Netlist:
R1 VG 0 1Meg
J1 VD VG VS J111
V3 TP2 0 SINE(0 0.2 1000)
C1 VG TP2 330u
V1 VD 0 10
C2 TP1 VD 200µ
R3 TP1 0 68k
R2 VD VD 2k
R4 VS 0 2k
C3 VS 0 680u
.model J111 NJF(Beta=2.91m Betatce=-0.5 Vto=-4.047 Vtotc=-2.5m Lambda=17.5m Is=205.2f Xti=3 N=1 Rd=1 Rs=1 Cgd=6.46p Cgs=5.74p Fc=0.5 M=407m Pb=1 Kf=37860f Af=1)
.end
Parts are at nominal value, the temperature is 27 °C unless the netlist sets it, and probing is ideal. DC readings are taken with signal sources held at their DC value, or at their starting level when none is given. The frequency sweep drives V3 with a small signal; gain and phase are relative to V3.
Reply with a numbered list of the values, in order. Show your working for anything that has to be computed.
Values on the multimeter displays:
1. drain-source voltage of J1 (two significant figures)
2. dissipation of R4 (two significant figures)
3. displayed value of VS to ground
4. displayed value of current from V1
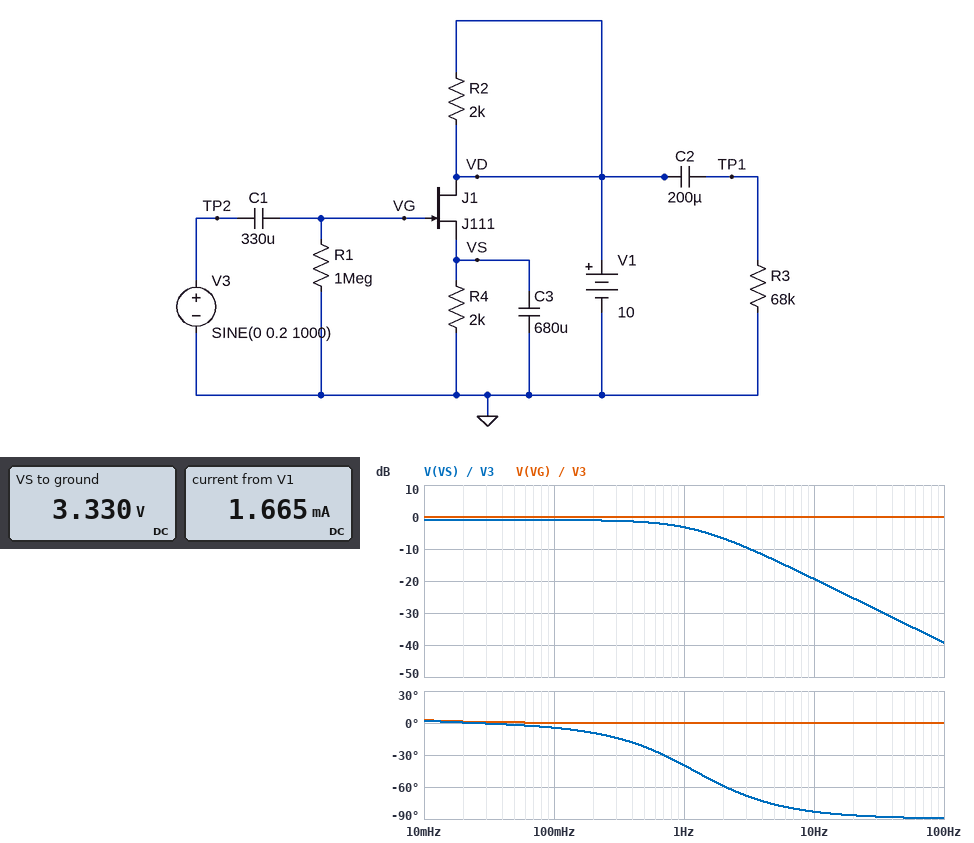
1. 10 V - 3.33 V = 6.7 V
2. (3.33 V)^2 / 2 kΩ = 5.5 mW
3. 3.330 V
4. 1.665 mA
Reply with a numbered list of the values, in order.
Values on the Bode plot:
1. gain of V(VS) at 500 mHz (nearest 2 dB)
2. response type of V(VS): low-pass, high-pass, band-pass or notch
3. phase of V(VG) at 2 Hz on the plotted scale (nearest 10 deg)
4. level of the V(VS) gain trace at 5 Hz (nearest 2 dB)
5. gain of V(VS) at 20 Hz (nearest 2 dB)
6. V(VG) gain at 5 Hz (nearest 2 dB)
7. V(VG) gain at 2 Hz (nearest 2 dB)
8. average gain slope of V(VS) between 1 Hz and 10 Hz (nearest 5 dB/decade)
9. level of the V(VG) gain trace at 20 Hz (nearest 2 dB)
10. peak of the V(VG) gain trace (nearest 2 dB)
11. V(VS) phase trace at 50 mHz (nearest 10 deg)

1. -2 dB
2. low-pass
3. 0 deg
4. -14 dB
5. -26 dB
6. 0 dB
7. 0 dB
8. -15 dB/decade
9. 0 dB
10. 0 dB
11. 0 deg
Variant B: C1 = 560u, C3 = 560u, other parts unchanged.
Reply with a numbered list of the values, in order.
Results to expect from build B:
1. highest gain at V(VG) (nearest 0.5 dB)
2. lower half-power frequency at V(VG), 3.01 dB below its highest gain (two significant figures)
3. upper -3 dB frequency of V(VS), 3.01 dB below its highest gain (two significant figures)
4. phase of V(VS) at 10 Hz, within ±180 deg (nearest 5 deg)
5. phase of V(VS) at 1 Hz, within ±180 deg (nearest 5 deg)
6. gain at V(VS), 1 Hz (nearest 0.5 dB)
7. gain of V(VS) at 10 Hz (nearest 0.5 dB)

1. 0 dB
2. 280 µHz
3. 1.5 Hz
4. -80 deg
5. -35 deg
6. -2.5 dB
7. -17.5 dB
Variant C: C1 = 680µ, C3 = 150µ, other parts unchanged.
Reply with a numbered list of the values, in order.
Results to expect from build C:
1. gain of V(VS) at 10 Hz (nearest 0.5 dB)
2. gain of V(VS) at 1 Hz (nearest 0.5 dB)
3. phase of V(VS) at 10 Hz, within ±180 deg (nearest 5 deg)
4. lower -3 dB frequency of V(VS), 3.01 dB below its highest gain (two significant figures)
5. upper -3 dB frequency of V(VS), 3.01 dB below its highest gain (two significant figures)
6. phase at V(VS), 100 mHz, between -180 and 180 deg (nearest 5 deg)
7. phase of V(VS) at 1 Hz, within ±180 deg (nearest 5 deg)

1. -7.5 dB
2. -1.0 dB
3. -60 deg
4. 230 µHz
5. 5.5 Hz
6. 0 deg
7. -10 deg
